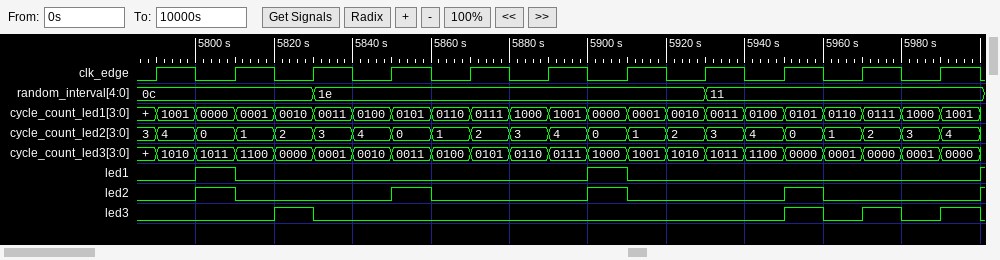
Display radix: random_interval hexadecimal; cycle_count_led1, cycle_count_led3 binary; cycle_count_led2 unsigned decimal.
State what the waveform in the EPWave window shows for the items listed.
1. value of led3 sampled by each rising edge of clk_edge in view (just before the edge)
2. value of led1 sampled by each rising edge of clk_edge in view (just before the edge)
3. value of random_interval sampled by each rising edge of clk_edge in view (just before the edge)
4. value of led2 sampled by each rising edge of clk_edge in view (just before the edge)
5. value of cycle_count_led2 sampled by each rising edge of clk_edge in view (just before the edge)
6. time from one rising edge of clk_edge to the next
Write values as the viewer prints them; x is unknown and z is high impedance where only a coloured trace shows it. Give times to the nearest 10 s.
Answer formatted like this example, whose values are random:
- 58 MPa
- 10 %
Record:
- 0 0 1 0 0 0 0 0 0 0 0
- 0 1 0 0 0 0 1 0 0 0 0
- 0c, 0c, 0c, 1e, 1e, 1e, 1e, 1e, 11, 11, 11
- 0 1 0 0 0 0 1 0 0 0 0
- 3, 0, 2, 4, 1, 3, 0, 2, 4, 1, 3
- 20 s
